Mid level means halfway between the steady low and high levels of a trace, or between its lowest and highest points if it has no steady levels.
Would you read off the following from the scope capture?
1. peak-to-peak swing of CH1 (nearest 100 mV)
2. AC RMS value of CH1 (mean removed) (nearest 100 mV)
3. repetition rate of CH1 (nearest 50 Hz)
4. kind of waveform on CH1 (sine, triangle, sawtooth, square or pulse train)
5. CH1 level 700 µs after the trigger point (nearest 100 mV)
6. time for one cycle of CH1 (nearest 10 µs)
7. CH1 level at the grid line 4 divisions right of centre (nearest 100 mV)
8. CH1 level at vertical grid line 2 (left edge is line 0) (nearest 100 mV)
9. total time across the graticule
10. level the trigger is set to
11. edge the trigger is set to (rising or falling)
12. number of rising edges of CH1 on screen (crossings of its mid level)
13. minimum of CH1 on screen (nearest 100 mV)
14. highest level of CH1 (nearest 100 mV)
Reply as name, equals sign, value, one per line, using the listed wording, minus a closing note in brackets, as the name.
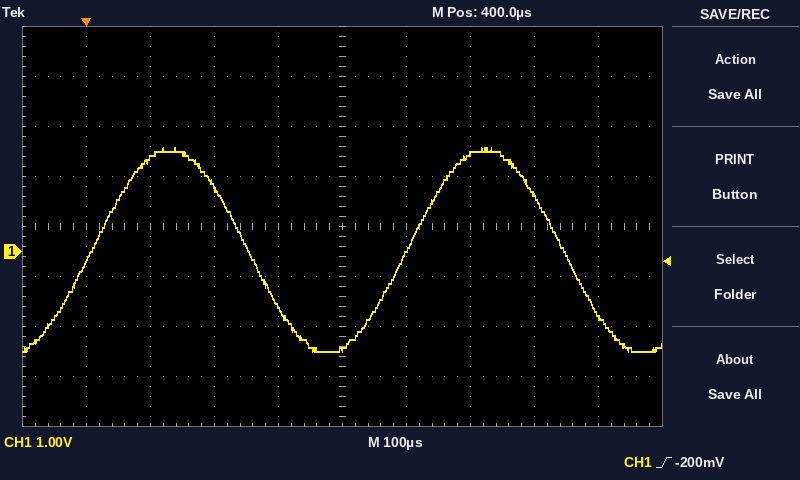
peak-to-peak swing of CH1 = 4.1 V
AC RMS value of CH1 (mean removed) = 1.4 V
repetition rate of CH1 = 2.05 kHz
kind of waveform on CH1 = sine
CH1 level 700 µs after the trigger point = 1.1 V
time for one cycle of CH1 = 490 µs
CH1 level at the grid line 4 divisions right of centre = -1.3 V
CH1 level at vertical grid line 2 (left edge is line 0) = 1.8 V
total time across the graticule = 1 ms
level the trigger is set to = -200 mV
edge the trigger is set to = rising
number of rising edges of CH1 on screen = 2
minimum of CH1 on screen = -2.0 V
highest level of CH1 = 2.1 V
